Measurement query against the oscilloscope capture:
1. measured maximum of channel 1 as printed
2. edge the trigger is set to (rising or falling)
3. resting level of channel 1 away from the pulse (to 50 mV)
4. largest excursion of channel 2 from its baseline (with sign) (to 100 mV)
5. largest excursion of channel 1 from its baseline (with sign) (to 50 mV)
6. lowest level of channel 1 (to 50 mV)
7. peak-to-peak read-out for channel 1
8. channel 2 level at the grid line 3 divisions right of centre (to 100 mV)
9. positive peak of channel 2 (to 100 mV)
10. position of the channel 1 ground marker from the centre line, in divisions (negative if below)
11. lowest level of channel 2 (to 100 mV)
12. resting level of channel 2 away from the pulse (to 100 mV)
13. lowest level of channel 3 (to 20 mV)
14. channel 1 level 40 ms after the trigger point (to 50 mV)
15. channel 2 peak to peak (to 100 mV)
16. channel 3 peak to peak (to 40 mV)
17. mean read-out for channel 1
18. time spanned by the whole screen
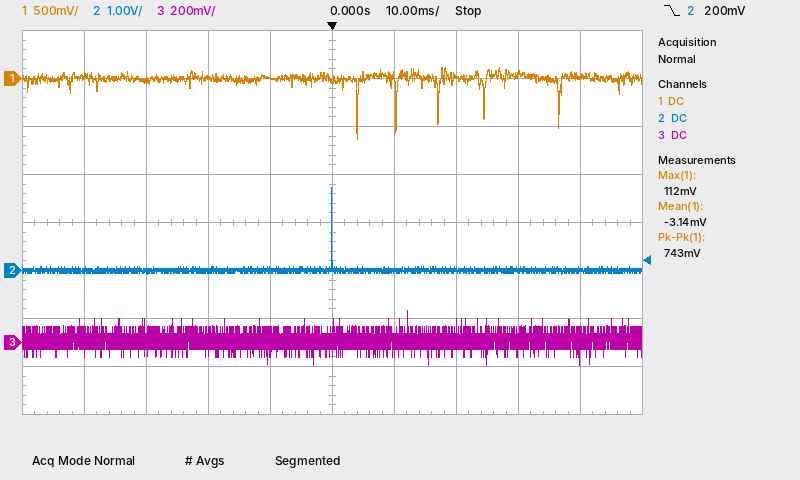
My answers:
112 mV
falling
0 mV
+1.7 V
-650 mV
-650 mV
743 mV
0.0 V
1.7 V
+3.0 div
-100 mV
0.0 V
-100 mV
0 mV
1.8 V
240 mV
-3.14 mV
100 ms
